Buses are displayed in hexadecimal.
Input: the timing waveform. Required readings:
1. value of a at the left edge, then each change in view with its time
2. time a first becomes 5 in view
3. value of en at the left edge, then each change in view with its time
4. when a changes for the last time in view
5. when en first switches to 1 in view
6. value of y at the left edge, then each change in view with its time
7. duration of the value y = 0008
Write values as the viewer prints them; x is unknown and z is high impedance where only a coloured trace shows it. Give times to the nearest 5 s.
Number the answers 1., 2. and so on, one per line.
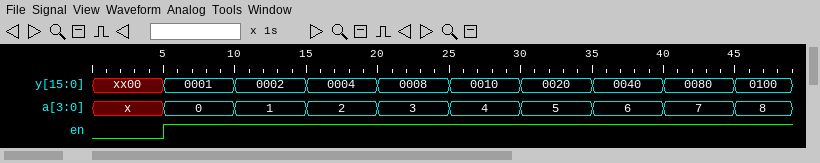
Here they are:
1. x, 0 at 5 s, 1 at 10 s, 2 at 15 s, 3 at 20 s, 4 at 25 s, 5 at 30 s, 6 at 35 s, 7 at 40 s, 8 at 45 s
2. 30 s
3. 0, 1 at 5 s
4. 45 s
5. 5 s
6. xx00, 0001 at 5 s, 0002 at 10 s, 0004 at 15 s, 0008 at 20 s, 0010 at 25 s, 0020 at 30 s, 0040 at 35 s, 0080 at 40 s, 0100 at 45 s
7. 5 s
